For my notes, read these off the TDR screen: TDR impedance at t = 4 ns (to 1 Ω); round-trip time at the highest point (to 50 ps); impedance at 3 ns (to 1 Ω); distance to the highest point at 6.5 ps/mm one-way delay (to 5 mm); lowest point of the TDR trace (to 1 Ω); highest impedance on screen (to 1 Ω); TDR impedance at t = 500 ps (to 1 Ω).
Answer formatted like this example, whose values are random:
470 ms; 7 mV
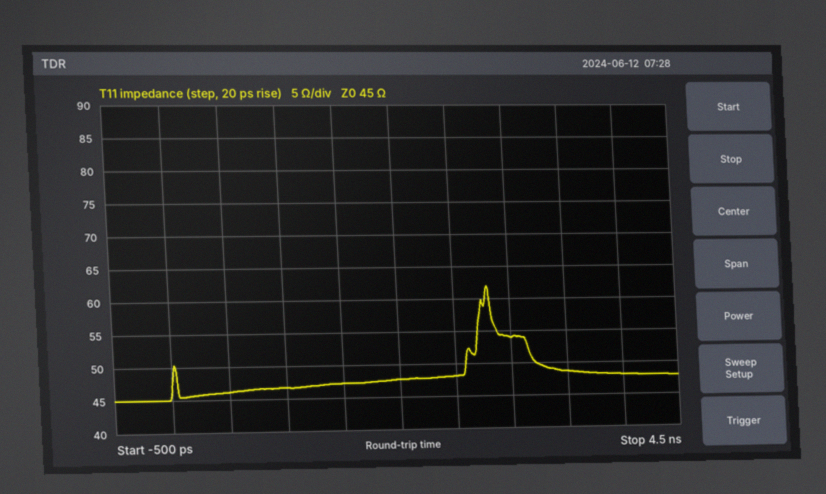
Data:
48 Ω; 2.80 ns; 54 Ω; 215 mm; 45 Ω; 62 Ω; 46 Ω
